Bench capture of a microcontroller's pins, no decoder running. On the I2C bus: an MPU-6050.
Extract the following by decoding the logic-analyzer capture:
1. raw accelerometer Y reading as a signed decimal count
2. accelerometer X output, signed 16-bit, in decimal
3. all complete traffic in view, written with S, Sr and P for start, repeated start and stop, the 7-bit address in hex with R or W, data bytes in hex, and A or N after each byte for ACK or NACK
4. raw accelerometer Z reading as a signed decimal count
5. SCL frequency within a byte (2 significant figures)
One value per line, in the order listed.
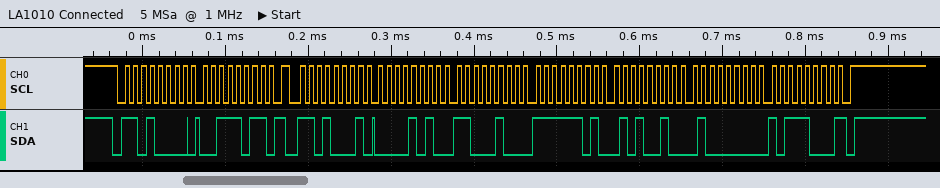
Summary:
-686
2756
S 68W A 3B A Sr 68R A 0A A C4 A FD A 52 A 40 A B8 N P
16568
100 kHz
